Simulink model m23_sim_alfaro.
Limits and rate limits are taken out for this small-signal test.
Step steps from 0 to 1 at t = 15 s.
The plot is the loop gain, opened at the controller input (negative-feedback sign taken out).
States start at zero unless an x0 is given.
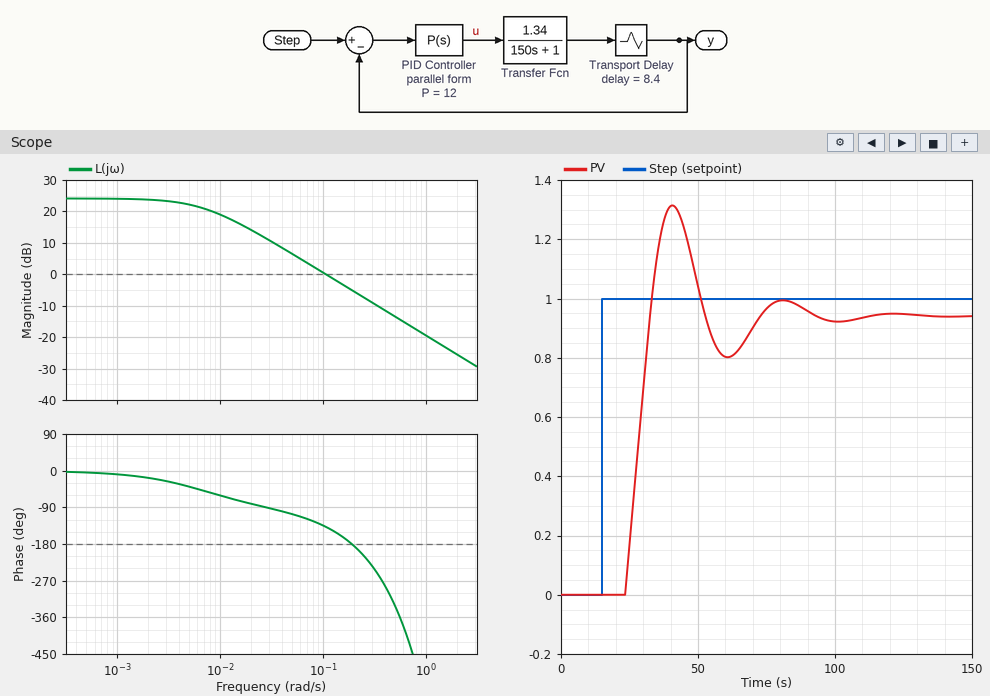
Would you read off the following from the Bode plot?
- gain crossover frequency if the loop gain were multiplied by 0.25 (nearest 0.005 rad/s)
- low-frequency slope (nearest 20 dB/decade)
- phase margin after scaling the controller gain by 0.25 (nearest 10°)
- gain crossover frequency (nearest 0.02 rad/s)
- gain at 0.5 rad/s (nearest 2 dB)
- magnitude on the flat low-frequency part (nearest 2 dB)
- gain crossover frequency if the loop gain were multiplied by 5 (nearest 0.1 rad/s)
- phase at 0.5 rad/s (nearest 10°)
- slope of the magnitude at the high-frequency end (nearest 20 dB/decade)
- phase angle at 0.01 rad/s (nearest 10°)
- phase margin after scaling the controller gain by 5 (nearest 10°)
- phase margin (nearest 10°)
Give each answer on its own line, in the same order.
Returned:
0.025 rad/s
0 dB/decade
90°
0.10 rad/s
-14 dB
24 dB
0.5 rad/s
-330°
-20 dB/decade
-60°
-170°
40°
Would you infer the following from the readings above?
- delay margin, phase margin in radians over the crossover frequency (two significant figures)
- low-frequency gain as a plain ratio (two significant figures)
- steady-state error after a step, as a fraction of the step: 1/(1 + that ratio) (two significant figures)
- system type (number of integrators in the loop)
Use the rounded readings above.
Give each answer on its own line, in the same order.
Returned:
7.0 s
16
0.059
0
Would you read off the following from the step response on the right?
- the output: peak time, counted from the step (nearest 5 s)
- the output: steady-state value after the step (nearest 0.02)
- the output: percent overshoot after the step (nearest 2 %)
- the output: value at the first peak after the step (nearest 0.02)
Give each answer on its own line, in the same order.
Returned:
25 s
0.94
40 %
1.32
